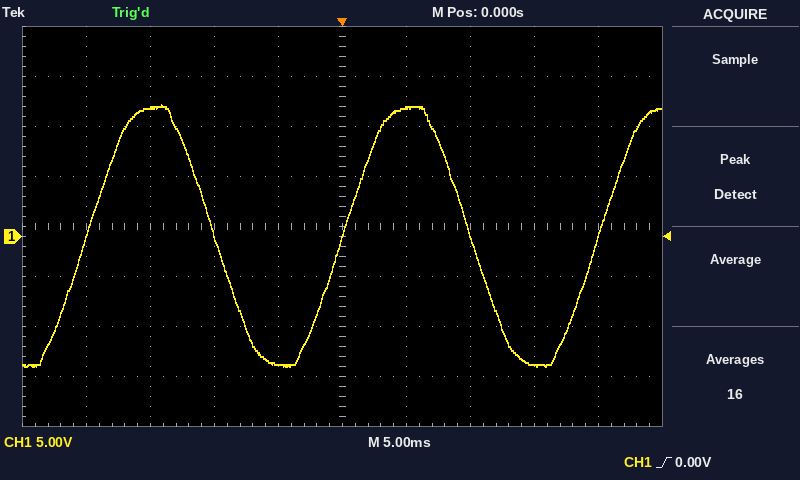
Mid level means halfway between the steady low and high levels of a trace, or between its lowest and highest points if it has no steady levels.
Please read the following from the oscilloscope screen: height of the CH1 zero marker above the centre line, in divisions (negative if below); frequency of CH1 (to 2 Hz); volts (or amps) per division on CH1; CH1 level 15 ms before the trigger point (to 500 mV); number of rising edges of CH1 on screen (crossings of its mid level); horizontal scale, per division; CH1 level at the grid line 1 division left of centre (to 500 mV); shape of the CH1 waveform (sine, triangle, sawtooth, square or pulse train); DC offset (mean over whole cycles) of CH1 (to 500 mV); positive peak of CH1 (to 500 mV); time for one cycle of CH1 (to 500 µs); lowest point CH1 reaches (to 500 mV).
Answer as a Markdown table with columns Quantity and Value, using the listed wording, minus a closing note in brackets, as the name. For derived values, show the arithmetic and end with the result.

| Quantity | Value |
|---|---|
| height of the CH1 zero marker above the centre line, in divisions | -0.2 div |
| frequency of CH1 | 1 / 20.0 ms ≈ 50 Hz |
| volts (or amps) per division on CH1 | 5 V |
| CH1 level 15 ms before the trigger point | 13.0 V |
| number of rising edges of CH1 on screen | 3 |
| horizontal scale, per division | 5 ms |
| CH1 level at the grid line 1 division left of centre | -13.0 V |
| shape of the CH1 waveform | sine |
| DC offset (mean over whole cycles) of CH1 | (13.0 V + (-13.0 V)) / 2 ≈ 0.0 V |
| positive peak of CH1 | 13.0 V |
| time for one cycle of CH1 | 20.0 ms |
| lowest point CH1 reaches | -13.0 V |
